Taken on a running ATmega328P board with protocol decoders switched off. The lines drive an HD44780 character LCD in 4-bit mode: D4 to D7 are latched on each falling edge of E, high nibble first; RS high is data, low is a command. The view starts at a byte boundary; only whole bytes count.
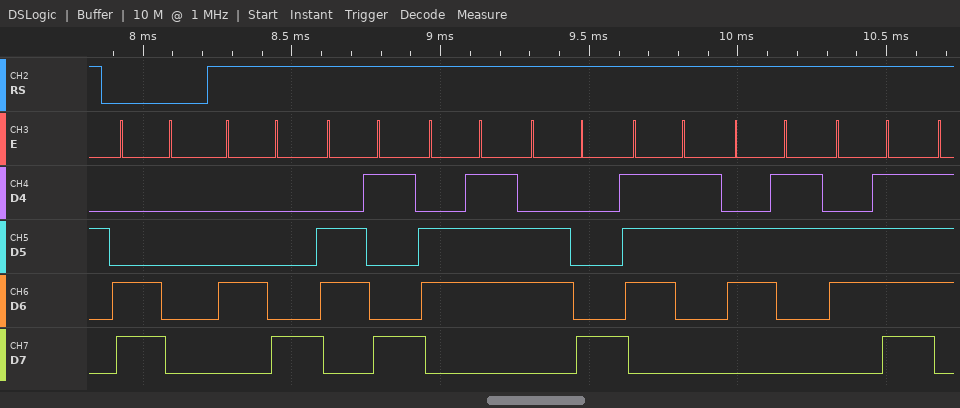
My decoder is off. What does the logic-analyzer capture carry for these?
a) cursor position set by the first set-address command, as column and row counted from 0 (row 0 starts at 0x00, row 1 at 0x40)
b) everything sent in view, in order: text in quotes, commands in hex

column 0, row 1
0xC0 "Highsco"
